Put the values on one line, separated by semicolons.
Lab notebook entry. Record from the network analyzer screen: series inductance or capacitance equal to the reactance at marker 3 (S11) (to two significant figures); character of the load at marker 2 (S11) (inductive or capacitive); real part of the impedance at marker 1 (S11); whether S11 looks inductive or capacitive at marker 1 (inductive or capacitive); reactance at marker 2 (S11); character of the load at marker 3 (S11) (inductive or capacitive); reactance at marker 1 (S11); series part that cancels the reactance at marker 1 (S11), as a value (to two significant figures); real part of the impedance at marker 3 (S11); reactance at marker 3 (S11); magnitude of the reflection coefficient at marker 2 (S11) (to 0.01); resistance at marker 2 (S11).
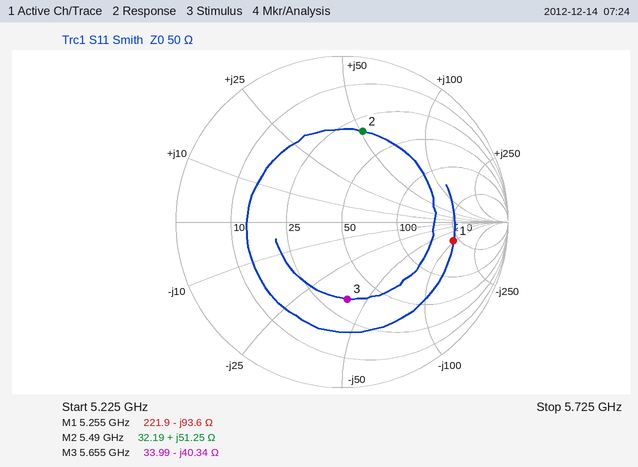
700 fF; inductive; 221.9 Ω; capacitive; +51.25 Ω; capacitive; -93.6 Ω; 2.8 nH; 33.99 Ω; -40.34 Ω; 0.56; 32.19 Ω
